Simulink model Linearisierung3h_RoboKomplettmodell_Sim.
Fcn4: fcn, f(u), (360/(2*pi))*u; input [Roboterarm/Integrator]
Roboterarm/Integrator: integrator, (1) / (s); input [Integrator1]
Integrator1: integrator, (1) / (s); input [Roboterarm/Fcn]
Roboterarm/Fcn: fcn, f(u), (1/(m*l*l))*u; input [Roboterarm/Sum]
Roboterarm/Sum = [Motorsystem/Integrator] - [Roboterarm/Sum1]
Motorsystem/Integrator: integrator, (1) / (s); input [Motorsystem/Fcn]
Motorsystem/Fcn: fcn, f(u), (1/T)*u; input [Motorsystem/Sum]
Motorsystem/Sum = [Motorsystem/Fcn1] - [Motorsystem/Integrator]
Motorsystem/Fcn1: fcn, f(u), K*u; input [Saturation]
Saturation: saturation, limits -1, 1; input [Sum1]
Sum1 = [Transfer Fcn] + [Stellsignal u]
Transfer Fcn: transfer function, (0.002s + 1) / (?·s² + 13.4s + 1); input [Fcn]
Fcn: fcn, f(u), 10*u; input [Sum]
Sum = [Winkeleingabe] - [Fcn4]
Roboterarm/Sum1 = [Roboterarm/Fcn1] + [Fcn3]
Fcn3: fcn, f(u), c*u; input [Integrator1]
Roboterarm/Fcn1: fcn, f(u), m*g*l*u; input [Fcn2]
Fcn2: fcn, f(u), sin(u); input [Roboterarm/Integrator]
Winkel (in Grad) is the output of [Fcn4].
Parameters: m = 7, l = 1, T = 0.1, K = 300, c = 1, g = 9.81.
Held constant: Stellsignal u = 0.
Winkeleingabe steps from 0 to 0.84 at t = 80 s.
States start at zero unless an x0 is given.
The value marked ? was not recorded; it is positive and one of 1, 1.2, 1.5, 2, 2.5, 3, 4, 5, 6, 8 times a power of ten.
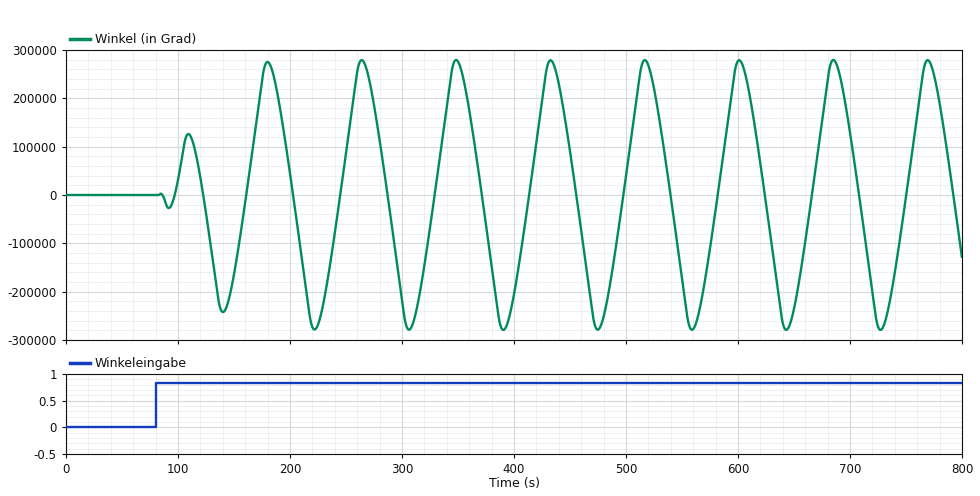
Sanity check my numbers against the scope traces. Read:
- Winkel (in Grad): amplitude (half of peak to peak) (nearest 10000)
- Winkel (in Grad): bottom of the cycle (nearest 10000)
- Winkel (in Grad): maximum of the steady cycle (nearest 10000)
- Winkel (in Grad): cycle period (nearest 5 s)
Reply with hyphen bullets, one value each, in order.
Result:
- 280000
- -280000
- 280000
- 85 s
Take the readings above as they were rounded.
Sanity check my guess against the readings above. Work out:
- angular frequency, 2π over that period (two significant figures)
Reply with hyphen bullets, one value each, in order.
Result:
- 0.074 rad/s
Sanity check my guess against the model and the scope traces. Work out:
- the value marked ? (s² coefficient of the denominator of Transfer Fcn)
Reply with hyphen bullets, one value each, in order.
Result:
- 80
